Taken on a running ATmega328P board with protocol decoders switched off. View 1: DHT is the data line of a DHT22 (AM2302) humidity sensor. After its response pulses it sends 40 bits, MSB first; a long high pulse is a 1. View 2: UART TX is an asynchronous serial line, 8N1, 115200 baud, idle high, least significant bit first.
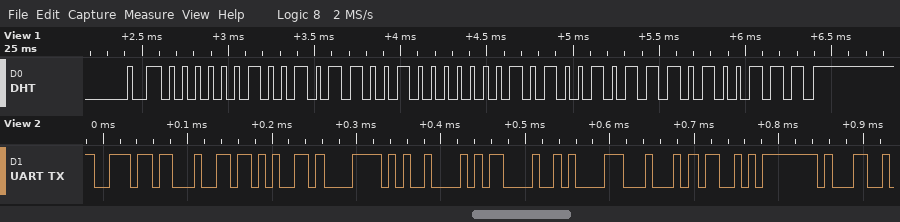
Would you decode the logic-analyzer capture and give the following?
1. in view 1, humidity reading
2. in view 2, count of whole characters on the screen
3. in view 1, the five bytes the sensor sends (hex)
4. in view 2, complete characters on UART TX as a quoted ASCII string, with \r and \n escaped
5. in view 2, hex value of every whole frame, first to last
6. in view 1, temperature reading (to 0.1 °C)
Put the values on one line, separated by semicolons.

60.1 %; 10; 02 59 01 4B A7; "ndex\t\r\nDS1"; 6E 64 65 78 09 0D 0A 44 53 31; 33.1 °C
